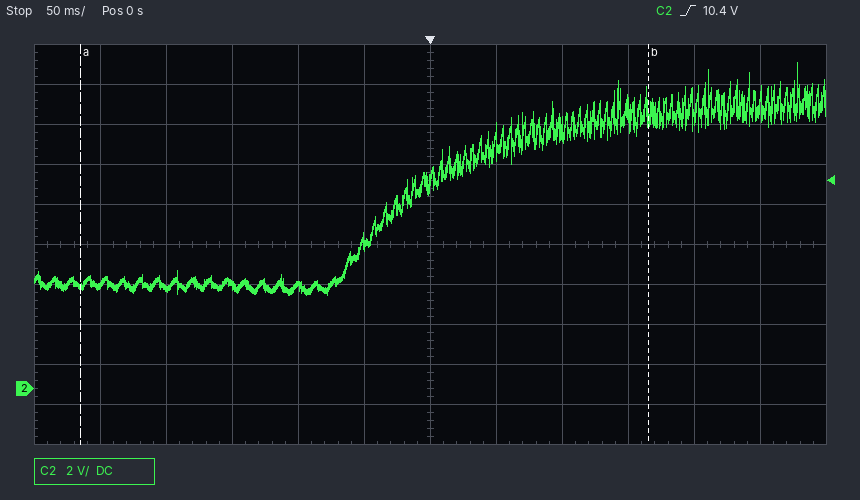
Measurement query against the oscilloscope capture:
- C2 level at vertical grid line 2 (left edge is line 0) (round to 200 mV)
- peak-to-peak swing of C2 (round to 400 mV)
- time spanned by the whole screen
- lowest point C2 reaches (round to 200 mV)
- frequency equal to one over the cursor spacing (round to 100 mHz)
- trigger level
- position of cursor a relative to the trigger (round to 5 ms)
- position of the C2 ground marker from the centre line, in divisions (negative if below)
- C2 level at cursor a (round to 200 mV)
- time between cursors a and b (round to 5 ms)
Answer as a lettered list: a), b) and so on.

a) 5.0 V
b) 11.6 V
c) 600 ms
d) 4.8 V
e) 2.3 Hz
f) 10.4 V
g) -265 ms
h) -3.6 div
i) 5.2 V
j) 430 ms
